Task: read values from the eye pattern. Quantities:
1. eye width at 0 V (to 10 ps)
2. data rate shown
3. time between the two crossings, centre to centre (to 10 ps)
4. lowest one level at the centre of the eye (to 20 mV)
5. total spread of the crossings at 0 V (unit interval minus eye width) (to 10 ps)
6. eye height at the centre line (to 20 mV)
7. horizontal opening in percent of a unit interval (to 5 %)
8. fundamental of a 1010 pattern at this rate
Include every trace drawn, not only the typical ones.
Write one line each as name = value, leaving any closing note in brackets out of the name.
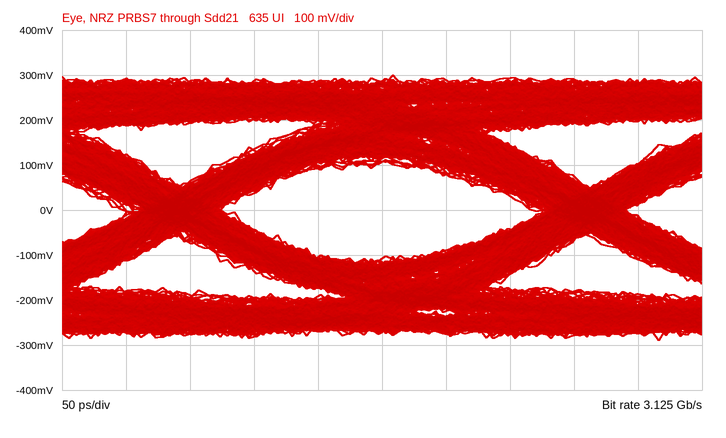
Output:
eye width at 0 V = 240 ps
data rate shown = 3.125 Gb/s
time between the two crossings, centre to centre = 320 ps
lowest one level at the centre of the eye = 100 mV
total spread of the crossings at 0 V (unit interval minus eye width) = 80 ps
eye height at the centre line = 220 mV
horizontal opening in percent of a unit interval = 75 %
fundamental of a 1010 pattern at this rate = 1.5625 GHz
